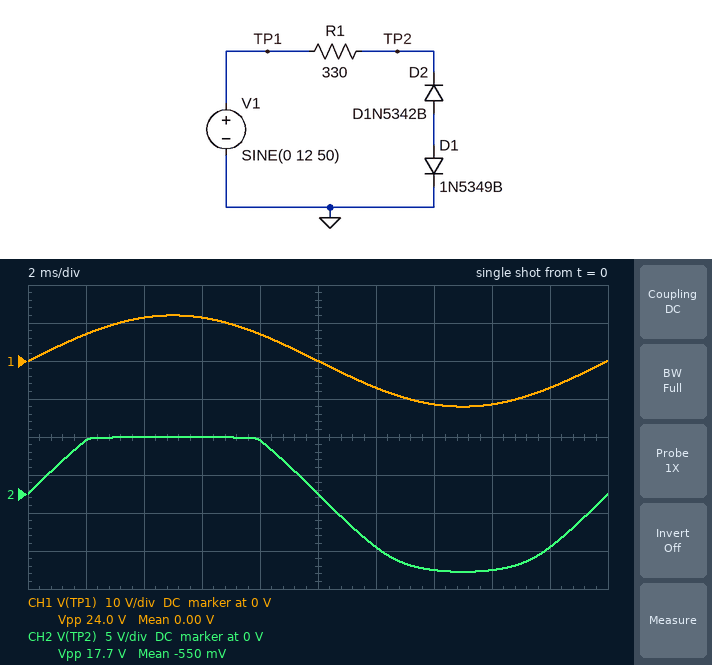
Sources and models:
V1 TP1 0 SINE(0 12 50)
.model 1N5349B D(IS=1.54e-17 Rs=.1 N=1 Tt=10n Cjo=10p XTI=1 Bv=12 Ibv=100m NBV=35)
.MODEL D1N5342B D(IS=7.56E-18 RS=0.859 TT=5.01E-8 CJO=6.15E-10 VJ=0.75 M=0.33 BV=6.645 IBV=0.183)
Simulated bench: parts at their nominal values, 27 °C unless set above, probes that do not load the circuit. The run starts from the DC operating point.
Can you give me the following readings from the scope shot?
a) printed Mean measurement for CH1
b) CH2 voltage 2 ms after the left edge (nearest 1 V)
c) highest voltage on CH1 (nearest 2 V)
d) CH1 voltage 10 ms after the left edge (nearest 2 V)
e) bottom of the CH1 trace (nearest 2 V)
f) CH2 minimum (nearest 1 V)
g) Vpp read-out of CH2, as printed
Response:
0.00 V
7 V
12 V
0 V
-12 V
-10 V
17.7 V
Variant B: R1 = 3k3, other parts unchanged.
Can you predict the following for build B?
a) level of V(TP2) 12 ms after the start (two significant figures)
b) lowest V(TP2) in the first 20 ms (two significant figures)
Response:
-6.7 V
-8.7 V
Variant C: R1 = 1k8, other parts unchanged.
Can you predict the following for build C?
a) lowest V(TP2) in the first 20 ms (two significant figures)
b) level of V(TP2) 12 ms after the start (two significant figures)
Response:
-9.1 V
-6.8 V
